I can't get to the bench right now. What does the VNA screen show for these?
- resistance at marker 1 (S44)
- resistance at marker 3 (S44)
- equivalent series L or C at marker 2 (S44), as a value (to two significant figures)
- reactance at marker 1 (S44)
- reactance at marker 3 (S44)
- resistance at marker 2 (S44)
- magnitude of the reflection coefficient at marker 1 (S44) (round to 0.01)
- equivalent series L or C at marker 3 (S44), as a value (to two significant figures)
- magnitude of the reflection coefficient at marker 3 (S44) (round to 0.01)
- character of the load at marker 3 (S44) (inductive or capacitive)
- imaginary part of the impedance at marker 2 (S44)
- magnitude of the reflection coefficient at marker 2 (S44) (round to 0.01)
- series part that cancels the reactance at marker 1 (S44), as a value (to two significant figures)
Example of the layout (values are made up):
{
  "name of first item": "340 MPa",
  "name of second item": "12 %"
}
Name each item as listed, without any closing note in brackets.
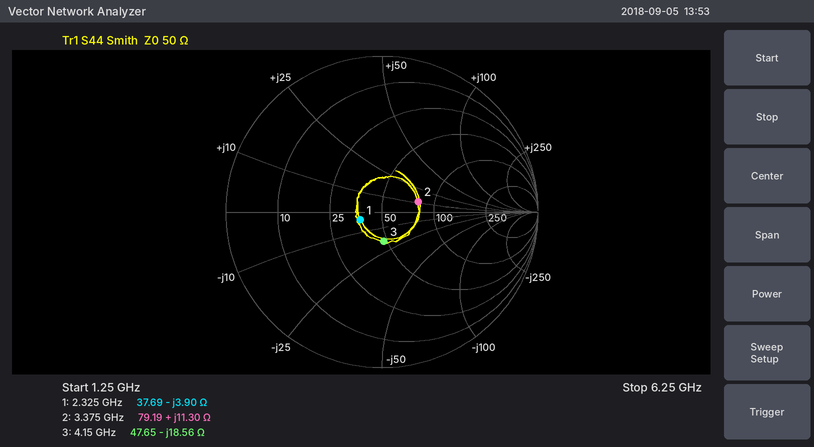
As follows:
{
  "resistance at marker 1": "37.69 Ω",
  "resistance at marker 3": "47.65 Ω",
  "equivalent series L or C at marker 2 (S44), as a value": "530 pH",
  "reactance at marker 1": "-3.90 Ω",
  "reactance at marker 3": "-18.56 Ω",
  "resistance at marker 2": "79.19 Ω",
  "magnitude of the reflection coefficient at marker 1 (S44)": "0.15",
  "equivalent series L or C at marker 3 (S44), as a value": "2.1 pF",
  "magnitude of the reflection coefficient at marker 3 (S44)": "0.19",
  "character of the load at marker 3 (S44)": "capacitive",
  "imaginary part of the impedance at marker 2": "+11.30 Ω",
  "magnitude of the reflection coefficient at marker 2 (S44)": "0.24",
  "series part that cancels the reactance at marker 1 (S44), as a value": "270 pH"
}
